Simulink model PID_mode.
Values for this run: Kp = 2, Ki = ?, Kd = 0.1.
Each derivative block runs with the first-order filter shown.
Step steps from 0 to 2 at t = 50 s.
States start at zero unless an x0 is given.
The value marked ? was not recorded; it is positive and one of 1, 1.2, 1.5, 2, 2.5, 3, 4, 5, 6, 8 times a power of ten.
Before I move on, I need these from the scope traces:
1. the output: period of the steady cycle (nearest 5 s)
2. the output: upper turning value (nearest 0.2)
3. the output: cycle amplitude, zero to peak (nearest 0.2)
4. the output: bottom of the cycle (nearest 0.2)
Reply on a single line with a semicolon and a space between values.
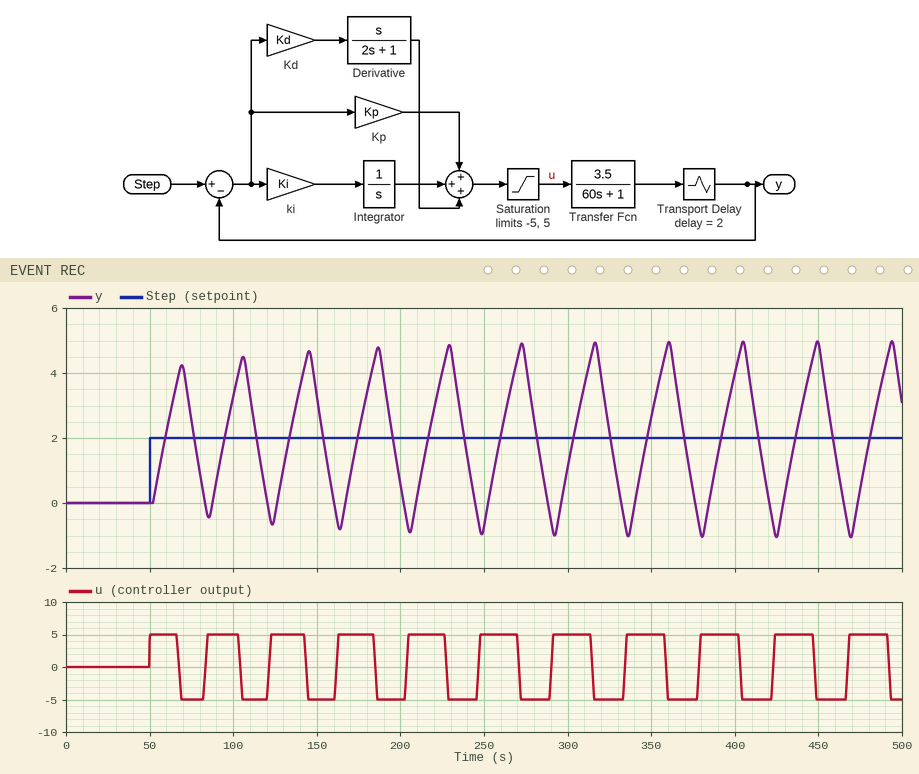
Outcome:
45 s; 5.0; 3.0; -1.0
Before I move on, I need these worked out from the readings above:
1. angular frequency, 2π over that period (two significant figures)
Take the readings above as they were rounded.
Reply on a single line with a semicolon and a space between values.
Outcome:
0.14 rad/s
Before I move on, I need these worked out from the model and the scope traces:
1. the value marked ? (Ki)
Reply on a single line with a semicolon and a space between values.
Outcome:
1.5
